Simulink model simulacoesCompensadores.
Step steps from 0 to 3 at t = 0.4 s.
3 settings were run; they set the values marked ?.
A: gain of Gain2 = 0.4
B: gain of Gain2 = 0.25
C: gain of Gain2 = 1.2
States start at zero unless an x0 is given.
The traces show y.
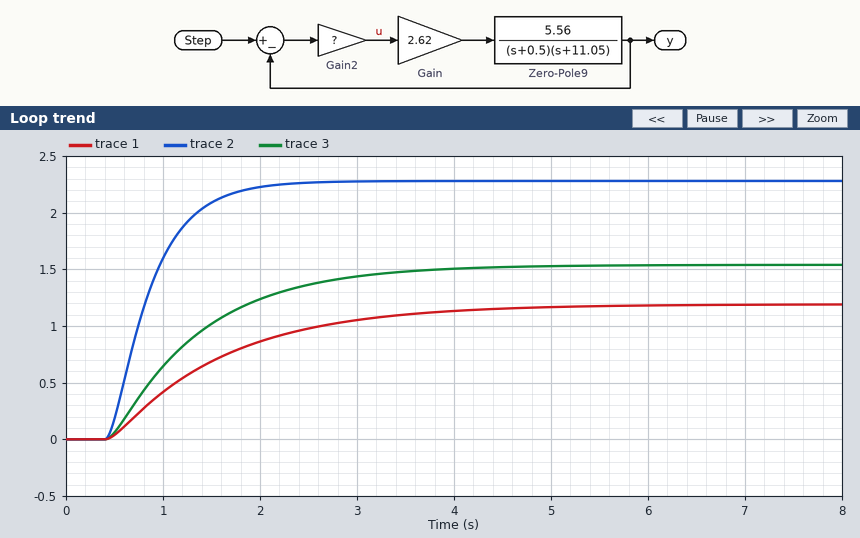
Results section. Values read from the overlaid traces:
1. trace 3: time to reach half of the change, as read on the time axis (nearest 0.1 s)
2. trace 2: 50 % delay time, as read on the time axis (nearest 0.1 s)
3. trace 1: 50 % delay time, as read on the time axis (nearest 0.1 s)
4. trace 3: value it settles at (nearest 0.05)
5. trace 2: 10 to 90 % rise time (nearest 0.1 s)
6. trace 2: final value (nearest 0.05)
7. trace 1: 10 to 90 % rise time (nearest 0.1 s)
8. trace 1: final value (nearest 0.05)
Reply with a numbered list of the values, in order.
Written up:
1. 1.1 s
2. 0.8 s
3. 1.3 s
4. 1.55
5. 0.9 s
6. 2.30
7. 2.6 s
8. 1.20
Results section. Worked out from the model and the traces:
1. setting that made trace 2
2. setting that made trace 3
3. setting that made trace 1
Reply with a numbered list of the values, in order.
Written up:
1. C
2. A
3. B
